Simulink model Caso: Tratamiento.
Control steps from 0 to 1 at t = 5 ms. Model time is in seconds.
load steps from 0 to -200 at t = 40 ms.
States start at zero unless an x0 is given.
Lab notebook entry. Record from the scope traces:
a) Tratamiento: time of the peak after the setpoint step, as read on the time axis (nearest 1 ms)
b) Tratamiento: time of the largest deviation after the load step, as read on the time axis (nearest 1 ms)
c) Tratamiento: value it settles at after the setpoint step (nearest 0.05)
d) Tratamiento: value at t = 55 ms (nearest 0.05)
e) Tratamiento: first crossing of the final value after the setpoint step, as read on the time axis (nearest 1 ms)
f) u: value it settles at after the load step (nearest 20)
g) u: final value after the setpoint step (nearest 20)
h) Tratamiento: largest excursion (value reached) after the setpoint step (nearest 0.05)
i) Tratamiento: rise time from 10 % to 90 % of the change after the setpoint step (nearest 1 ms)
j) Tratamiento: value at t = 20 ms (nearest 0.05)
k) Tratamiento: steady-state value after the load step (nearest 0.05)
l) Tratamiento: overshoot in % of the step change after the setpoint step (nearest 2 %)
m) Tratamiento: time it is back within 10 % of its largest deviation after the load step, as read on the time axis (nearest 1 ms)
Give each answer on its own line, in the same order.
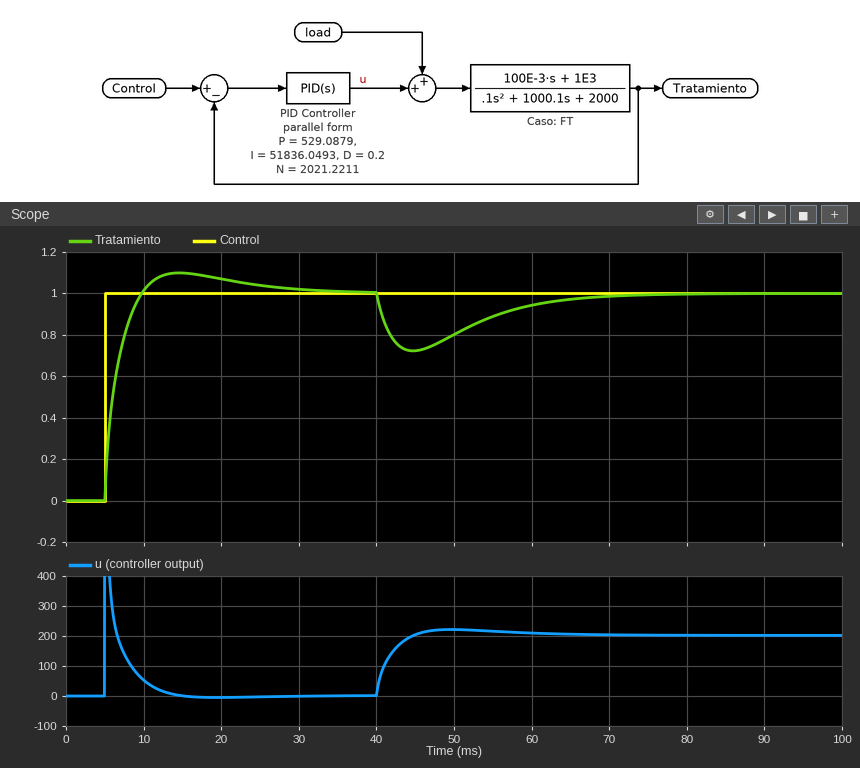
15 ms
45 ms
1.00
0.90
10 ms
200
0
1.10
3 ms
1.05
1.00
10 %
65 ms
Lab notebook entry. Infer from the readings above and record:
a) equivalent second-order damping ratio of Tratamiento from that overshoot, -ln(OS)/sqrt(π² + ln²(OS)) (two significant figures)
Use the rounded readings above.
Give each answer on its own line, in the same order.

0.59
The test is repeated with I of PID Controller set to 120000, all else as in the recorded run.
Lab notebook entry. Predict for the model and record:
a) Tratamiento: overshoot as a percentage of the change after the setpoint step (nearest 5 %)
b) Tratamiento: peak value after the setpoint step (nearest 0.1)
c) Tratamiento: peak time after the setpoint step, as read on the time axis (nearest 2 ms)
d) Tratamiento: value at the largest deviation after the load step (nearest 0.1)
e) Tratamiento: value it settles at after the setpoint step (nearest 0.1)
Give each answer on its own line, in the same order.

15 %
1.2
12 ms
0.8
1.0
